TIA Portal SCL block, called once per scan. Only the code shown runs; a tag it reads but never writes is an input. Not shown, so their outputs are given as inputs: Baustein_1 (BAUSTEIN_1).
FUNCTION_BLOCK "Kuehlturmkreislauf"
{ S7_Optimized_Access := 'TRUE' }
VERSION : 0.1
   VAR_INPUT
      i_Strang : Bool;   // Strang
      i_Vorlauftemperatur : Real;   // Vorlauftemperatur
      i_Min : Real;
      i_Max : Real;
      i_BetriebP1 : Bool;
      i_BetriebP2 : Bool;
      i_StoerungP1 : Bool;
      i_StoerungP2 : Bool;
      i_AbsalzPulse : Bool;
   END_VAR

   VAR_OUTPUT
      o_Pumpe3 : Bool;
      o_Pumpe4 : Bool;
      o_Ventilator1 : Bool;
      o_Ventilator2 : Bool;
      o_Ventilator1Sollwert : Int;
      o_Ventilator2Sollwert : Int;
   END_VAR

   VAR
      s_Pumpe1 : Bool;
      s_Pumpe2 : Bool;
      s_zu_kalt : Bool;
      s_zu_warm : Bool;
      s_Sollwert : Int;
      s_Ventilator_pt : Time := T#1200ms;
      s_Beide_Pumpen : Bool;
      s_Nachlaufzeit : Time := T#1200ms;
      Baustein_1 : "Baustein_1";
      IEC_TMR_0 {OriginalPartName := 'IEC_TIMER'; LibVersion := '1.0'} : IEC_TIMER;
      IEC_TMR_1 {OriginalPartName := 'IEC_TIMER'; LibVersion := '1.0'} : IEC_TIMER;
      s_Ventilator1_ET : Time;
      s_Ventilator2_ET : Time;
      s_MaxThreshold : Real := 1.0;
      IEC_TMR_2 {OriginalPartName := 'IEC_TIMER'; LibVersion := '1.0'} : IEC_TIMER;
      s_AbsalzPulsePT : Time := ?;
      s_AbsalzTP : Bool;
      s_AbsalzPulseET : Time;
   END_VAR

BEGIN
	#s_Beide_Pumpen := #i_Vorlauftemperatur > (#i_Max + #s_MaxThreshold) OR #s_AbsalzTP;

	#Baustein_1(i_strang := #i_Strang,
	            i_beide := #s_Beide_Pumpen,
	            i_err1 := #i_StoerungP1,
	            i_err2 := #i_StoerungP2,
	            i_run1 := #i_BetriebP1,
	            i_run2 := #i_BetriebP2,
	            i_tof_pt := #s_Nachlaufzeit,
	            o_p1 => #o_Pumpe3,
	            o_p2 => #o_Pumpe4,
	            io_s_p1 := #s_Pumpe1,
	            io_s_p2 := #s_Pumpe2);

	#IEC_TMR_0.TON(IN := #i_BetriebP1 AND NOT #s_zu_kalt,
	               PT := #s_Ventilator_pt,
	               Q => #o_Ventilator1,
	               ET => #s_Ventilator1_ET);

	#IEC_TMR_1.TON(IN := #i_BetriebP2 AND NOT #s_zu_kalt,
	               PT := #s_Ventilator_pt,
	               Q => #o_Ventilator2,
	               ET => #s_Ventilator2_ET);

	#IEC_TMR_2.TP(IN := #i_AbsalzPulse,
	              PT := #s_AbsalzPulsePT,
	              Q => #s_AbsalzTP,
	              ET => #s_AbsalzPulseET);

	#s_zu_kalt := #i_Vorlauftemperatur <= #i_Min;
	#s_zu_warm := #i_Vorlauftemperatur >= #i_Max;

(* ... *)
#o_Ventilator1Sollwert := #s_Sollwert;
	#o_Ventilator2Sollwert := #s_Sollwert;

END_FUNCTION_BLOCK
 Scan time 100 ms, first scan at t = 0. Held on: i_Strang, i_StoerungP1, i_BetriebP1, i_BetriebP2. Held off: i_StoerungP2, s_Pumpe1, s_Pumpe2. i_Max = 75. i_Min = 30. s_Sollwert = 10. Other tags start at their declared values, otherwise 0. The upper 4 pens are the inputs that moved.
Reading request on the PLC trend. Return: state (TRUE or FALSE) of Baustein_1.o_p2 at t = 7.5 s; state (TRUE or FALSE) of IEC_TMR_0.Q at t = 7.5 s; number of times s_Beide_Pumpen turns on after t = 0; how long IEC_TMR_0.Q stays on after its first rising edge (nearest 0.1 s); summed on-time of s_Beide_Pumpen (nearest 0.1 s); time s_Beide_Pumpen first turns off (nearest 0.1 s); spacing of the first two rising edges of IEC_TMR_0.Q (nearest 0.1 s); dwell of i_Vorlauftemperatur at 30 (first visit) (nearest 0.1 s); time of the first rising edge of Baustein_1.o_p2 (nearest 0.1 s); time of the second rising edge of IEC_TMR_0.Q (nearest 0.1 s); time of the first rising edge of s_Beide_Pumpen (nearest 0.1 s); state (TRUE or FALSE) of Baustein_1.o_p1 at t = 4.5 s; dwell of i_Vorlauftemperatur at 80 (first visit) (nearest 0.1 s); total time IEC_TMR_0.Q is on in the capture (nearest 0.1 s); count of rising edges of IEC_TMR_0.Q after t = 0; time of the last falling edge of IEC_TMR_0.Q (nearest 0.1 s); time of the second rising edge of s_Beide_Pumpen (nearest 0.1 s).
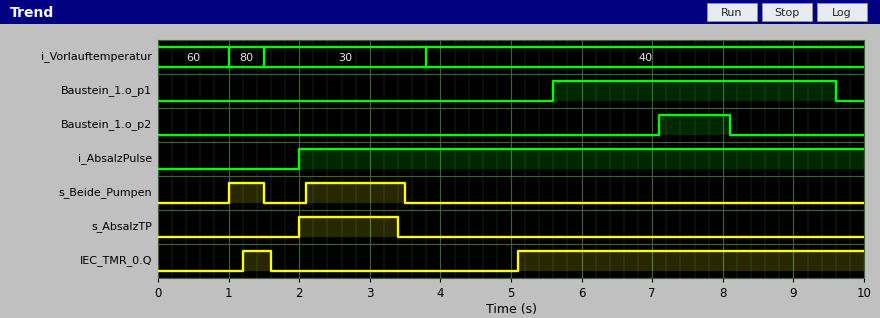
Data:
TRUE
TRUE
2
0.4 s
1.9 s
1.5 s
3.9 s
2.3 s
7.1 s
5.1 s
1.0 s
FALSE
0.5 s
5.3 s
2
1.6 s
2.1 s
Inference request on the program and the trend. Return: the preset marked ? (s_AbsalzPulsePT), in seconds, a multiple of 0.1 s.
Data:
1.4 s
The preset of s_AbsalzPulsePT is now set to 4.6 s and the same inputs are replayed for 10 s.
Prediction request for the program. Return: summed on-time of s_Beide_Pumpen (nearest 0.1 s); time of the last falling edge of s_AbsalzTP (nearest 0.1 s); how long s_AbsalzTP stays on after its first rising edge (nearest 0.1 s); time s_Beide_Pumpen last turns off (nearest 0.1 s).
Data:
5.1 s
6.6 s
4.6 s
6.7 s
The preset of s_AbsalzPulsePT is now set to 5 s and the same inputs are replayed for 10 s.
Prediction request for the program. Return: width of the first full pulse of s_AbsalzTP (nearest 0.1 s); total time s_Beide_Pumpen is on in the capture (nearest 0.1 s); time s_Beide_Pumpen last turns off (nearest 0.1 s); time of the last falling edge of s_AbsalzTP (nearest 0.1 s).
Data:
5.0 s
5.5 s
7.1 s
7.0 s
